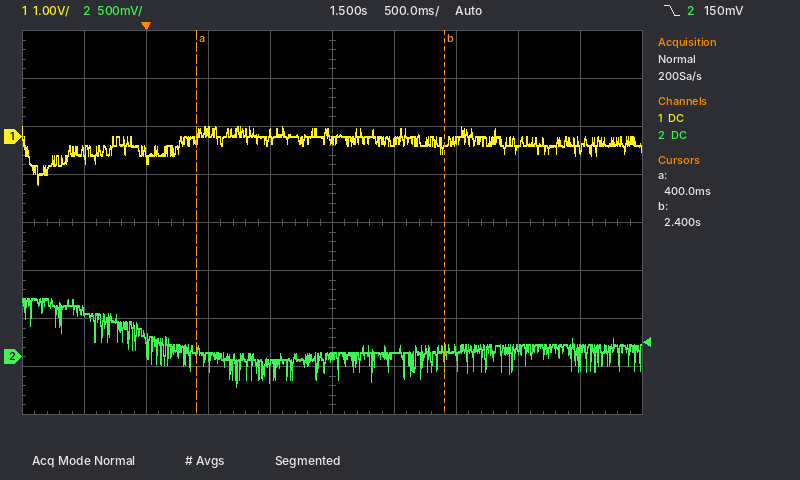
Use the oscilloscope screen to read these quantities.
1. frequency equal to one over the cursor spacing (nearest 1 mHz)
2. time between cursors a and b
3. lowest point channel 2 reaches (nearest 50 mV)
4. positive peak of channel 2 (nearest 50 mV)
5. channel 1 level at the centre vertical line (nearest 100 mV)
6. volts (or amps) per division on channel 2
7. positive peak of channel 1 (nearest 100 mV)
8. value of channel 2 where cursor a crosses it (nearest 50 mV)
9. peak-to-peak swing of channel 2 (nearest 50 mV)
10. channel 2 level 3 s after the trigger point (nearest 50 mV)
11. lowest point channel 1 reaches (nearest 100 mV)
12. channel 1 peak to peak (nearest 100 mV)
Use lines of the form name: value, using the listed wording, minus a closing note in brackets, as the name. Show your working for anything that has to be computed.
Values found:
frequency equal to one over the cursor spacing: 1 / 2.00 s ≈ 500 mHz
time between cursors a and b: 2.4 s − (400 ms) = 2.00 s
lowest point channel 2 reaches: -300 mV
positive peak of channel 2: 600 mV
channel 1 level at the centre vertical line: -100 mV
volts (or amps) per division on channel 2: 500 mV
positive peak of channel 1: 200 mV
value of channel 2 where cursor a crosses it: 50 mV
peak-to-peak swing of channel 2: 600 mV − (-300 mV) = 900 mV
channel 2 level 3 s after the trigger point: 100 mV
lowest point channel 1 reaches: -1.0 V
channel 1 peak to peak: 200 mV − (-1.0 V) = 1.2 V
